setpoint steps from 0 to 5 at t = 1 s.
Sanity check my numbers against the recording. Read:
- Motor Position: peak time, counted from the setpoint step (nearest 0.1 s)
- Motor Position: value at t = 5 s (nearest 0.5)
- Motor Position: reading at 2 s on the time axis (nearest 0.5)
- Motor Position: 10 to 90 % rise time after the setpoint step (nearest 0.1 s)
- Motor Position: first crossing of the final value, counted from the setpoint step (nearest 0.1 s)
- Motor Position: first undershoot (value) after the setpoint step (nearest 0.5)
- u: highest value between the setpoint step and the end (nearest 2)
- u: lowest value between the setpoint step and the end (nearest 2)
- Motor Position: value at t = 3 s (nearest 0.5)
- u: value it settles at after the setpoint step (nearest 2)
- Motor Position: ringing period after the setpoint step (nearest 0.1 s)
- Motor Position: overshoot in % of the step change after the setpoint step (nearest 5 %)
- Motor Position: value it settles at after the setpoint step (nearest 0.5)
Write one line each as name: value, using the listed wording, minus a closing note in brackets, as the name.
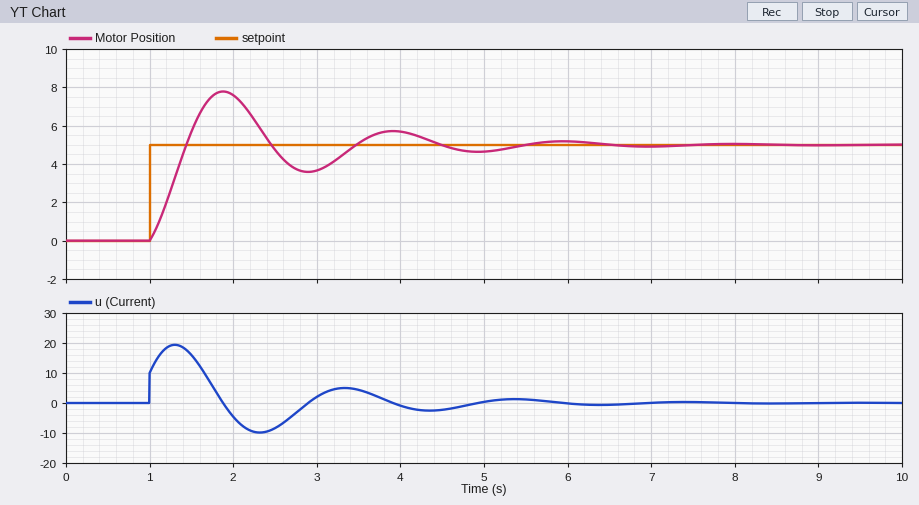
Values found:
Motor Position: peak time, counted from the setpoint step: 0.9 s
Motor Position: value at t = 5 s: 4.5
Motor Position: reading at 2 s on the time axis: 7.5
Motor Position: 10 to 90 % rise time after the setpoint step: 0.3 s
Motor Position: first crossing of the final value, counted from the setpoint step: 0.4 s
Motor Position: first undershoot (value) after the setpoint step: 3.5
u: highest value between the setpoint step and the end: 20
u: lowest value between the setpoint step and the end: -10
Motor Position: value at t = 3 s: 3.5
u: value it settles at after the setpoint step: 0
Motor Position: ringing period after the setpoint step: 2.0 s
Motor Position: overshoot in % of the step change after the setpoint step: 55 %
Motor Position: value it settles at after the setpoint step: 5.0
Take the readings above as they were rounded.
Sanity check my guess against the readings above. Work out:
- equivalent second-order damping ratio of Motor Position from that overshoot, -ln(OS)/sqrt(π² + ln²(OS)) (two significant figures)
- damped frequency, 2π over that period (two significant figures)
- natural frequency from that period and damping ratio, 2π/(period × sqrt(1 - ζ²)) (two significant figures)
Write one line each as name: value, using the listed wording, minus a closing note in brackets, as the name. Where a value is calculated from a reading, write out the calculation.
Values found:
equivalent second-order damping ratio of Motor Position from that overshoot, -ln(OS)/sqrt(π² + ln²(OS)): ln(0.55) = -0.598; 0.598 / sqrt(9.870 + 0.357) = 0.19
damped frequency, 2π over that period: 2π / 2 = 3.1 rad/s
natural frequency from that period and damping ratio, 2π/(period × sqrt(1 - ζ²)): 2π / (2 × sqrt(1 - 0.19²)) = 3.2 rad/s
